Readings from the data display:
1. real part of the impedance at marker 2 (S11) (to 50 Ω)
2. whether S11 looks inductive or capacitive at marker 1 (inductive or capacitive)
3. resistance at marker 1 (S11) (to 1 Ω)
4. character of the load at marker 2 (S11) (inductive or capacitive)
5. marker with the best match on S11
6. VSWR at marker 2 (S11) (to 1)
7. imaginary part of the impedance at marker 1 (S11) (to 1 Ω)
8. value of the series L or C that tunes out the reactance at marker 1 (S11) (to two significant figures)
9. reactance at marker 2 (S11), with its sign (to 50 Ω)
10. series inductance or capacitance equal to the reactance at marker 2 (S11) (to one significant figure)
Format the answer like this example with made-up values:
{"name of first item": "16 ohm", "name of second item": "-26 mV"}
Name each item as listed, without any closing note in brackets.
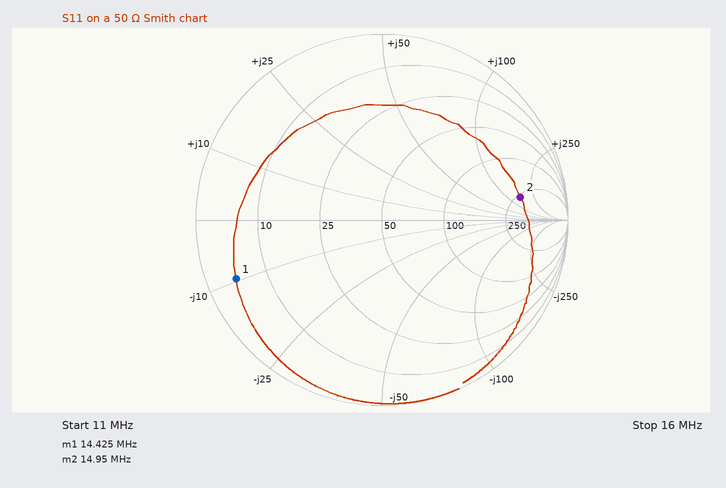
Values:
{"real part of the impedance at marker 2 (S11)": "250 Ω", "whether S11 looks inductive or capacitive at marker 1": "capacitive", "resistance at marker 1 (S11)": "4 Ω", "character of the load at marker 2 (S11)": "inductive", "marker with the best match on S11": "marker 2", "VSWR at marker 2 (S11)": "7", "imaginary part of the impedance at marker 1 (S11)": "-10 Ω", "value of the series L or C that tunes out the reactance at marker 1 (S11)": "110 nH", "reactance at marker 2 (S11), with its sign": "+150 Ω", "series inductance or capacitance equal to the reactance at marker 2 (S11)": "2 µH"}
